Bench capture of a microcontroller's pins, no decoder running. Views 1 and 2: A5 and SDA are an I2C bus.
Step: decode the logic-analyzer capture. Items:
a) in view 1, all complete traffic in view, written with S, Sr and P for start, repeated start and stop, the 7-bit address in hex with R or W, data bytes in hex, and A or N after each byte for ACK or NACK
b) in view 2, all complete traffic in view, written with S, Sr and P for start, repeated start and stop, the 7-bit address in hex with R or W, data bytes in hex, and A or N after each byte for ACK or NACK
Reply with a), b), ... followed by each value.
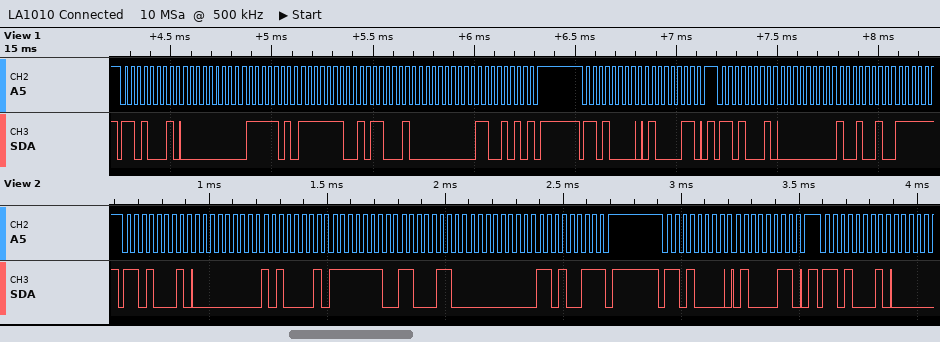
a) S 68R A 00 A 7D A FE A B1 A 00 A CA N P S 68W A 43 A P S 68R A 00 A 92 A
b) S 68R A 00 A A1 A FE A C6 A 00 A D3 N P S 68W A 43 A P S 68R A
